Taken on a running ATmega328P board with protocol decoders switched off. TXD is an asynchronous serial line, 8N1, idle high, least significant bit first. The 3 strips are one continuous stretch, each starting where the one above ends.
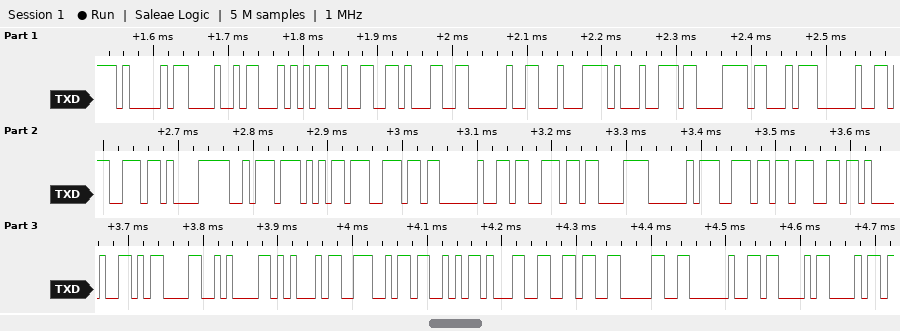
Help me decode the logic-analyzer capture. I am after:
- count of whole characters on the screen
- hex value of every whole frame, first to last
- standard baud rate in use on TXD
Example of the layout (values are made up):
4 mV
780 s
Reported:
34
41 48 54 32 31 20 C4 91 C3 A3 20 73 E1 BA B5 6E 20 73 C3 A0 6E 67 21 0D 0A 45 4E 53 31 36 30 20 43 68
115200 baud
